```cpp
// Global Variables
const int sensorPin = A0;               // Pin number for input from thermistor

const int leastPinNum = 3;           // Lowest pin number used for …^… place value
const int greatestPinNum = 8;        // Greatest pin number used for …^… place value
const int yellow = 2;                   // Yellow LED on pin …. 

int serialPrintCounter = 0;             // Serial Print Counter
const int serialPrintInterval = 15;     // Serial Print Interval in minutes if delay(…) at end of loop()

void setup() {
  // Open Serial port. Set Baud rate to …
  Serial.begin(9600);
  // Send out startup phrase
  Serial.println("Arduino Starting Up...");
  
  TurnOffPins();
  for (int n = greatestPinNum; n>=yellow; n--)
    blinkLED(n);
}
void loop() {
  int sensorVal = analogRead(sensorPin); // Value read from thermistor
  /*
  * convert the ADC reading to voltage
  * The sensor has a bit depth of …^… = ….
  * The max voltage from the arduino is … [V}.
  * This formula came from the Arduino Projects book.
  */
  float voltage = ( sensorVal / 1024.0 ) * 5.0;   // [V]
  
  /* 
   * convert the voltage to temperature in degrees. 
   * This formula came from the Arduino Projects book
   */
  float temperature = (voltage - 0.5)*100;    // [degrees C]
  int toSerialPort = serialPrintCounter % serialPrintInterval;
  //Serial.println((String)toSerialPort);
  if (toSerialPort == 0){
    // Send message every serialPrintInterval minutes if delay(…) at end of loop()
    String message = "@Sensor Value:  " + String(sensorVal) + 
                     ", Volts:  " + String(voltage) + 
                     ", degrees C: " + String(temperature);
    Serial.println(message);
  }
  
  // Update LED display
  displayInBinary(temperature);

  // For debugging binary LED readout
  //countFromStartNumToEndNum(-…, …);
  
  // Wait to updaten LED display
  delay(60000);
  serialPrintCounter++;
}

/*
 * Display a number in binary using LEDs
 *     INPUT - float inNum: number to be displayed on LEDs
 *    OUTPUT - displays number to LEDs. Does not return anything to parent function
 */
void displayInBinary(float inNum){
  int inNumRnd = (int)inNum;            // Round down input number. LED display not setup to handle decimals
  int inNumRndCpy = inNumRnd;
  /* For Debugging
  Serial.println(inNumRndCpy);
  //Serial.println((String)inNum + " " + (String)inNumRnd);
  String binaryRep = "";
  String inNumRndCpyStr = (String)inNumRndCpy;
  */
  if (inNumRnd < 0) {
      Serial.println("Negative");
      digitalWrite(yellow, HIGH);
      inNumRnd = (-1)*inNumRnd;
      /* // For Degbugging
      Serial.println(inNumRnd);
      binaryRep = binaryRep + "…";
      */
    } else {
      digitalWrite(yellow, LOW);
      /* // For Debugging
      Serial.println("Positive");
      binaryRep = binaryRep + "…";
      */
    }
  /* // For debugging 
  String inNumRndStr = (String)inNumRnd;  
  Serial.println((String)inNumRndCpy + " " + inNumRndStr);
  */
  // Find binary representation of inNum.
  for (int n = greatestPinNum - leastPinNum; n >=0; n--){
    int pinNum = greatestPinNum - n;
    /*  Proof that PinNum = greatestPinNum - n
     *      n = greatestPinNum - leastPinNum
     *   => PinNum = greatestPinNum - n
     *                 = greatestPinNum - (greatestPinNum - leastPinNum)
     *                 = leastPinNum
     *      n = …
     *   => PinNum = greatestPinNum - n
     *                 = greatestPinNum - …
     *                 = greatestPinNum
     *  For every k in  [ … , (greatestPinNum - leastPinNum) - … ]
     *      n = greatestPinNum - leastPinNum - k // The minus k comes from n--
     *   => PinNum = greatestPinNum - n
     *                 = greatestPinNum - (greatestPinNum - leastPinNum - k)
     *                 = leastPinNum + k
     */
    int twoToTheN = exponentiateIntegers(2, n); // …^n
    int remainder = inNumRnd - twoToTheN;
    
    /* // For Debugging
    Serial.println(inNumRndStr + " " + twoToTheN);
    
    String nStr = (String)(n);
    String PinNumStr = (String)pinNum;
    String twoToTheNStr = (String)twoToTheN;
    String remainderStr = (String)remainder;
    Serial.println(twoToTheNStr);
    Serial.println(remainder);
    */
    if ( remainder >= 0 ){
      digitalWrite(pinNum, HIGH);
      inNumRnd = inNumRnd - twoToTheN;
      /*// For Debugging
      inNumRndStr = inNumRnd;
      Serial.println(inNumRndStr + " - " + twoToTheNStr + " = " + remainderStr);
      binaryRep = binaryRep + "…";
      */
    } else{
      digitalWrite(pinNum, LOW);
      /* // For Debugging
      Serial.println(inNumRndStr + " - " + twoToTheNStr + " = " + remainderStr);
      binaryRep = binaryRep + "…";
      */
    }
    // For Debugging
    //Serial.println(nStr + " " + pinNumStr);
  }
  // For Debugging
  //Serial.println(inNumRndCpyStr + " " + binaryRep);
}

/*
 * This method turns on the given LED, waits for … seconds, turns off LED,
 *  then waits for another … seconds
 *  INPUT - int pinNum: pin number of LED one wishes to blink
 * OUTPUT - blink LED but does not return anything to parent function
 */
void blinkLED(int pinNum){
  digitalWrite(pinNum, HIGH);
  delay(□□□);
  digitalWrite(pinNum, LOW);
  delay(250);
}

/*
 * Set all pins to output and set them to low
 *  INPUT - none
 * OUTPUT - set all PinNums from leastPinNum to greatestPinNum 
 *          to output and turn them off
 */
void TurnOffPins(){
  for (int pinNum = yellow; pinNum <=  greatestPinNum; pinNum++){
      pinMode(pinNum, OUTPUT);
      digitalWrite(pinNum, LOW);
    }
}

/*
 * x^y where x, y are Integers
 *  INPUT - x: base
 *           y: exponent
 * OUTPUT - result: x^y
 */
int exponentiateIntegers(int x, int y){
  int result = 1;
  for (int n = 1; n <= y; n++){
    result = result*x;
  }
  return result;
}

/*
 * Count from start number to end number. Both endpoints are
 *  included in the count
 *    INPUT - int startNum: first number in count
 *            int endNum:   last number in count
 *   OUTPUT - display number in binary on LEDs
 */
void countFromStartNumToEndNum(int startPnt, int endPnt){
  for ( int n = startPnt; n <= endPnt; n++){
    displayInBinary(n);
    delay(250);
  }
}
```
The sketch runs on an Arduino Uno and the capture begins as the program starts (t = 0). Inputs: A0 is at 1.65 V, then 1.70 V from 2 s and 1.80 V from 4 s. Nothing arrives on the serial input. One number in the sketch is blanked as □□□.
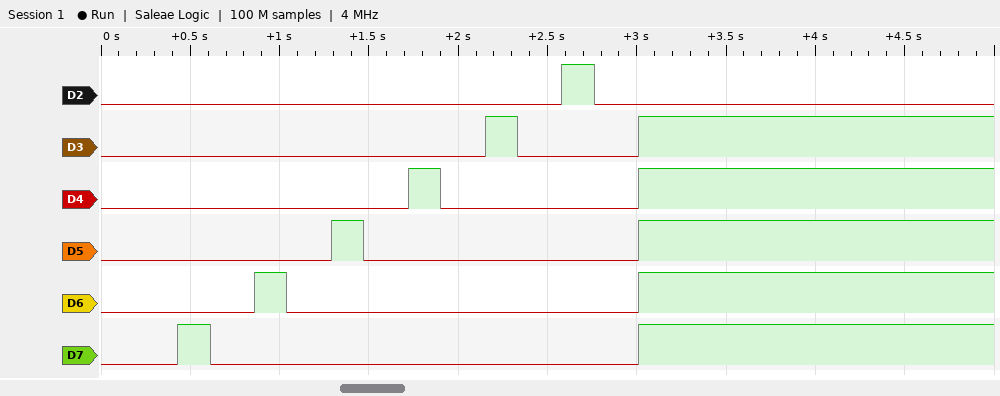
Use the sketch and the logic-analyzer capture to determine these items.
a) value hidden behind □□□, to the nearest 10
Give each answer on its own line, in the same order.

180
